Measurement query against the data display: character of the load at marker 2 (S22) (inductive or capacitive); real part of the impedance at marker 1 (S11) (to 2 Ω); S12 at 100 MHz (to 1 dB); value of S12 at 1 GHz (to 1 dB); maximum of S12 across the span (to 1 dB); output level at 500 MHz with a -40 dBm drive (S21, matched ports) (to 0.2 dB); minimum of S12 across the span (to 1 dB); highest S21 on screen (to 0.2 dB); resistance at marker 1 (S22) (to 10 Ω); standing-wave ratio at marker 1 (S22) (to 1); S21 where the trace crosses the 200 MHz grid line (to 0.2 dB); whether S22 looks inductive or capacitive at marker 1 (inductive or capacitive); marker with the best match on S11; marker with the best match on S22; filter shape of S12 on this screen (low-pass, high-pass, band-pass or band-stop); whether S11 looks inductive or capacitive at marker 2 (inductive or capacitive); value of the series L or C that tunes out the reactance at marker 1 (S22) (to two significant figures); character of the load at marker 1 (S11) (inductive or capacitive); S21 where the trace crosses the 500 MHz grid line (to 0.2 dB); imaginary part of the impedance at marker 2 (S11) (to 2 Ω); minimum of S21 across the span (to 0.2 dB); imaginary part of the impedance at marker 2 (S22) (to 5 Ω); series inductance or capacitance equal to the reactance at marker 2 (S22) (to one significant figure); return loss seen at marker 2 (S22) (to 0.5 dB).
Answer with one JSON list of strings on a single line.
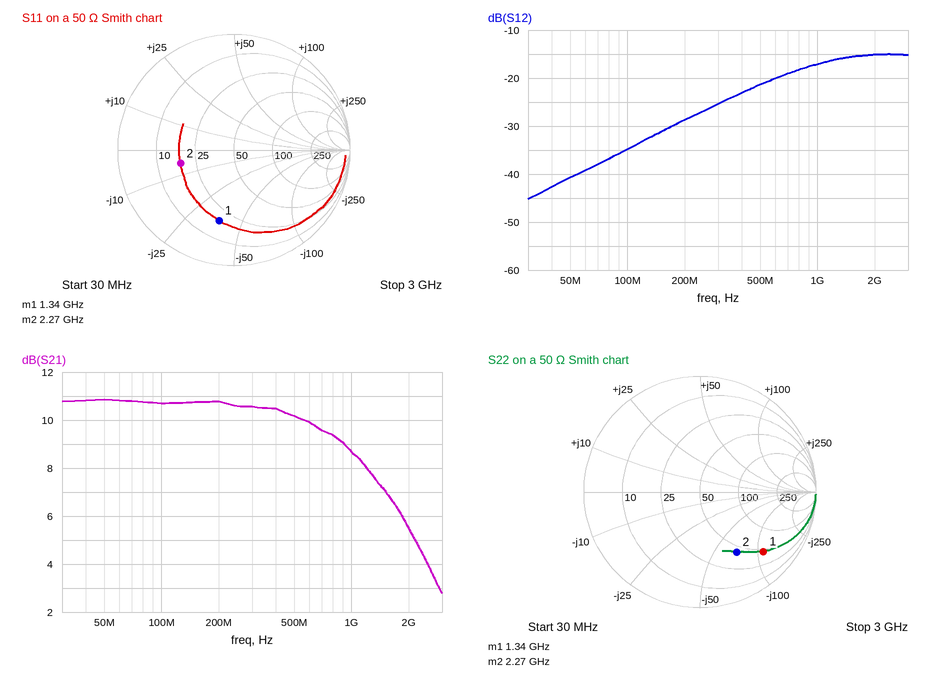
["capacitive", "18 Ω", "-35 dB", "-17 dB", "-15 dB", "-29.8 dBm", "-45 dB", "10.8 dB", "50 Ω", "7", "10.8 dB", "capacitive", "marker 2", "marker 2", "high-pass", "capacitive", "13 nH", "capacitive", "10.2 dB", "-6 Ω", "2.8 dB", "-70 Ω", "1.0 pF", "4.5 dB"]
